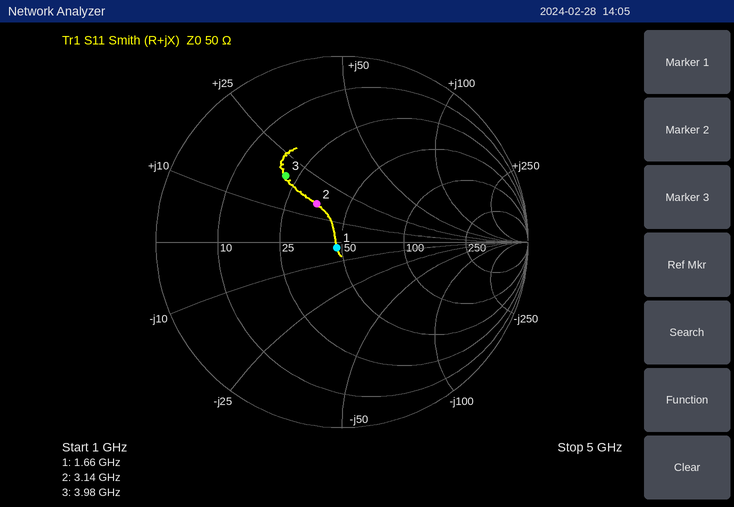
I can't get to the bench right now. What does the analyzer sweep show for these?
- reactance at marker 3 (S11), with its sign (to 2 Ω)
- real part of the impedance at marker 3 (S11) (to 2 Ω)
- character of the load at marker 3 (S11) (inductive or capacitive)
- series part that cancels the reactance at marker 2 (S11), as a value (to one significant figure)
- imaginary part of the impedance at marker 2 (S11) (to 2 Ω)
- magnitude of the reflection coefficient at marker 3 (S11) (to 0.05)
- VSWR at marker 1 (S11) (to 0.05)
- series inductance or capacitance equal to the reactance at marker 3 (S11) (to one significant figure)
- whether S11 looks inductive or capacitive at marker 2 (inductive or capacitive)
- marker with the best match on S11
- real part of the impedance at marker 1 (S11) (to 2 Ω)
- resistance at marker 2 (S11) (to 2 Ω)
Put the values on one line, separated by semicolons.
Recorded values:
+20 Ω; 22 Ω; inductive; 3 pF; +16 Ω; 0.45; 1.10; 800 pH; inductive; marker 1; 48 Ω; 36 Ω
